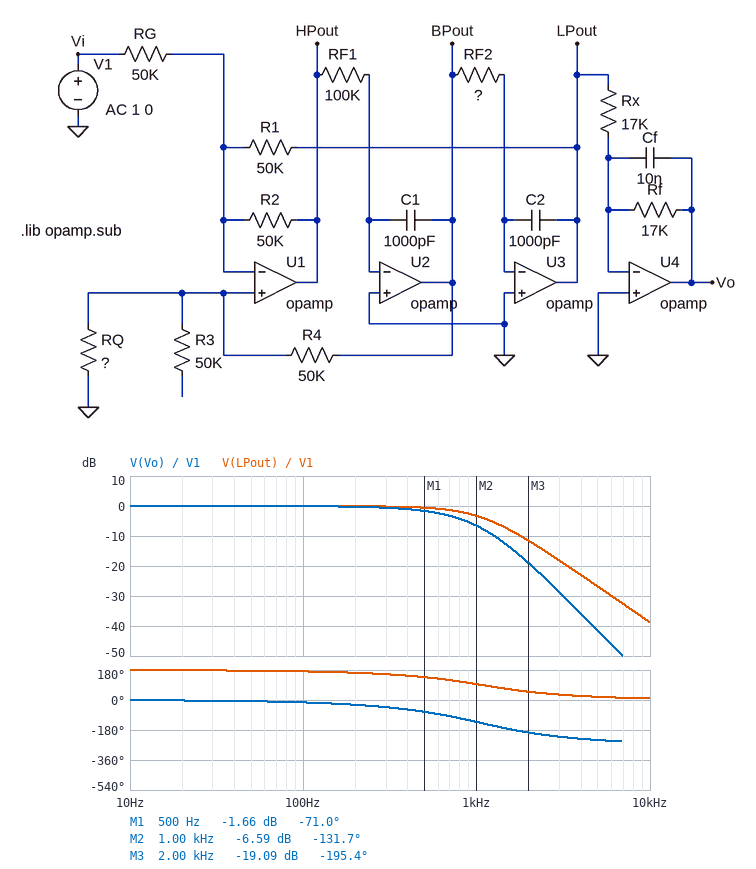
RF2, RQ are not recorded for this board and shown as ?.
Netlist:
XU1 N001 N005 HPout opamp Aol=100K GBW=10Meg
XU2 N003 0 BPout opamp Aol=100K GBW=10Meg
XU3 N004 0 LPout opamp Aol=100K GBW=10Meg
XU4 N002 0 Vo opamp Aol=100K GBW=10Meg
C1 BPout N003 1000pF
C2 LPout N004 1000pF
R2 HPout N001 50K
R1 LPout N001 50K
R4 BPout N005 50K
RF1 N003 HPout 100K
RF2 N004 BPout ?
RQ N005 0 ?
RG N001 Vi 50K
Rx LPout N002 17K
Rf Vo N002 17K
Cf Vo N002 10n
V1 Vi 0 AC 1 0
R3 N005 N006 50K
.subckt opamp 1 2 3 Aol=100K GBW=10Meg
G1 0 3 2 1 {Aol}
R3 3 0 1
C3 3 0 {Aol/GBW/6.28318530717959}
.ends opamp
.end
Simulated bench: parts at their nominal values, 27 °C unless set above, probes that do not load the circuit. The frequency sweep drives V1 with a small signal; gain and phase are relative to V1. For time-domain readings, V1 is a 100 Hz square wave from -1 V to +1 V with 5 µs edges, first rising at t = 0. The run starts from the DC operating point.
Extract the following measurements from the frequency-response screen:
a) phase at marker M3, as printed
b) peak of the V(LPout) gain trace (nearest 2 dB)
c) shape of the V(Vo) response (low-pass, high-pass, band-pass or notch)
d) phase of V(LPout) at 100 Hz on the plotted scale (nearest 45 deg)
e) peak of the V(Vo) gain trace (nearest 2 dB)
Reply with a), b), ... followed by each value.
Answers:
a) -195.4 deg
b) 0 dB
c) low-pass
d) 180 deg
e) 0 dB
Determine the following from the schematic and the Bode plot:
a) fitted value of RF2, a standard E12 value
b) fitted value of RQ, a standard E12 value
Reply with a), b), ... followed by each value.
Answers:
a) 220 kΩ
b) 27 kΩ
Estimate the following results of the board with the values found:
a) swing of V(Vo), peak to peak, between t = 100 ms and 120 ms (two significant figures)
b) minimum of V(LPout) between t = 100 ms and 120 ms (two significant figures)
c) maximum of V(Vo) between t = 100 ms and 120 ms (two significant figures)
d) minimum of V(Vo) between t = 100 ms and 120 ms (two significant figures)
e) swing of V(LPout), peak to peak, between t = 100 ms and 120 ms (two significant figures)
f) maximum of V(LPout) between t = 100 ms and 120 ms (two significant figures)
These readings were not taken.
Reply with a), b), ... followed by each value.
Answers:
a) 2.0 V
b) -1.0 V
c) 1.0 V
d) -1.0 V
e) 2.1 V
f) 1.0 V
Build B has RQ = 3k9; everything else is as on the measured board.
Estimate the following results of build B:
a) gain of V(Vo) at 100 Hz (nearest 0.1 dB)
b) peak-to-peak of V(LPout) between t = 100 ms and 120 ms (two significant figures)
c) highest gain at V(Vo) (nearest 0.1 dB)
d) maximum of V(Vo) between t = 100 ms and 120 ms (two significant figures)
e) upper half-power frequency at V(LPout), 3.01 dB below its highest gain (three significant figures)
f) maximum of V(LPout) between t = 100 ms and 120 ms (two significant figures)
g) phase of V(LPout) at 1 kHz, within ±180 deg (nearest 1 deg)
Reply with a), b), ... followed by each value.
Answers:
a) 0 dB
b) 4.4 V
c) 6.5 dB
d) 1.7 V
e) 1.21 kHz
f) 2.2 V
g) 114 deg
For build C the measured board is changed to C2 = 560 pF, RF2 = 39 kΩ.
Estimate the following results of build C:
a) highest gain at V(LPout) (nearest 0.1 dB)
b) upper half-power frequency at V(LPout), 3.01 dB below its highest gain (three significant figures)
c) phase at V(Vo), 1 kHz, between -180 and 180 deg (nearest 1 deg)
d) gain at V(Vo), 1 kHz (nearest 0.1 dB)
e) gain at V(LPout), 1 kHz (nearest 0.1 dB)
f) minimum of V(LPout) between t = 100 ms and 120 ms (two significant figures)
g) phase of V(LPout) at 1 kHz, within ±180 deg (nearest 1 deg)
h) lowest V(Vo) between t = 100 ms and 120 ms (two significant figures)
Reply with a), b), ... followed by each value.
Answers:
a) 6.5 dB
b) 3.96 kHz
c) -56 deg
d) -2.6 dB
e) 0.7 dB
f) -1.9 V
g) 171 deg
h) -1.0 V
